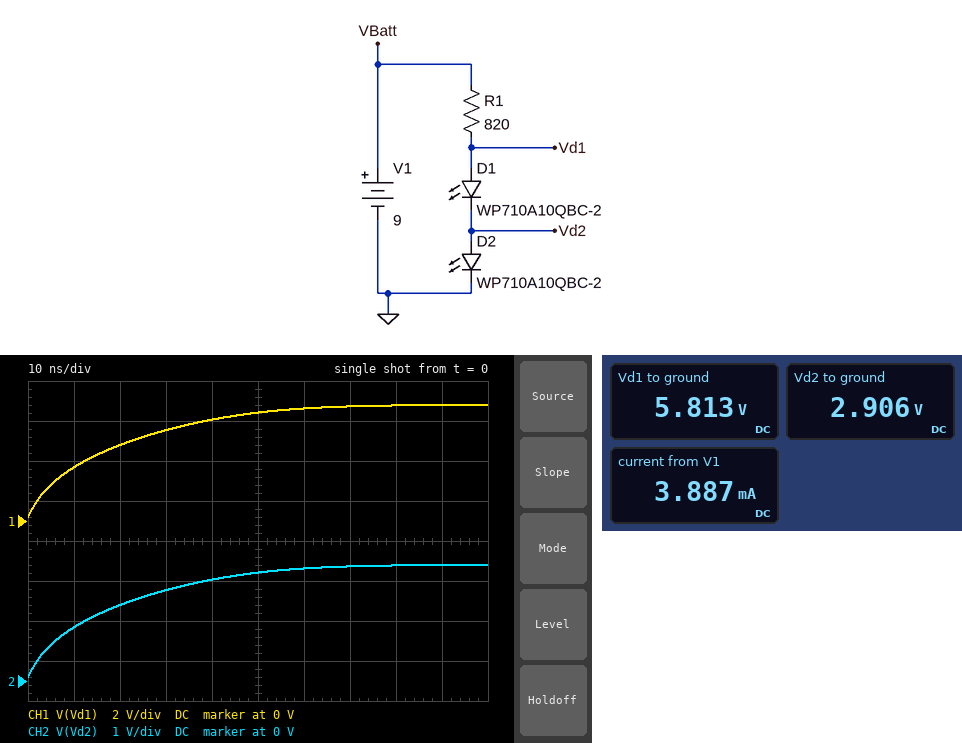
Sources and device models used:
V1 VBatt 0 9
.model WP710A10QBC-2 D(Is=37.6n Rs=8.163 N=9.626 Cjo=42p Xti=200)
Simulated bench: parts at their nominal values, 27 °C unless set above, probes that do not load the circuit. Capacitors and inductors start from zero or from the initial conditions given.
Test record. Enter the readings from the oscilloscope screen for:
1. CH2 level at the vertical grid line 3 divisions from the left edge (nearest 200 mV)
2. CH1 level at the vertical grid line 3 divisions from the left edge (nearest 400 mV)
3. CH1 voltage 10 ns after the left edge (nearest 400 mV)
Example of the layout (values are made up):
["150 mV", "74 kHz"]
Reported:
["2.2 V", "4.4 V", "2.8 V"]
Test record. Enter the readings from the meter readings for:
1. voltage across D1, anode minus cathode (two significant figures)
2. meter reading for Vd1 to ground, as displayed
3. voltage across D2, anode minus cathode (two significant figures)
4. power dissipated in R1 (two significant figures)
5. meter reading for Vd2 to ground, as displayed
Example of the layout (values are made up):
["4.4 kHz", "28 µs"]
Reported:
["2.9 V", "5.813 V", "2.9 V", "12 mW", "2.906 V"]
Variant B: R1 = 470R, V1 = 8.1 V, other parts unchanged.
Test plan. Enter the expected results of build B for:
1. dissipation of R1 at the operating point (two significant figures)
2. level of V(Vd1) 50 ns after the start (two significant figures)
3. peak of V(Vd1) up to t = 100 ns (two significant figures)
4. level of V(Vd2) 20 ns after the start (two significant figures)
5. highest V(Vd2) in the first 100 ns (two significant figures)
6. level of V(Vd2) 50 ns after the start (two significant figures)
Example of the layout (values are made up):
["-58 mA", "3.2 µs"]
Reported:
["10 mW", "5.8 V", "5.9 V", "2.3 V", "3.0 V", "2.9 V"]
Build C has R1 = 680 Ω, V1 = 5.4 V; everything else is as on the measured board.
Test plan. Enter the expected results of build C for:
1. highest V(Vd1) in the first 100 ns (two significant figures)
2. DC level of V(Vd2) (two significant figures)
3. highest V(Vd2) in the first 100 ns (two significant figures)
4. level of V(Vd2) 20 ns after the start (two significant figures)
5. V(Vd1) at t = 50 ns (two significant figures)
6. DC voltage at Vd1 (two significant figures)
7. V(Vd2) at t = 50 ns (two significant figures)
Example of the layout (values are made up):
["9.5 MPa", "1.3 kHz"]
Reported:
["4.7 V", "2.5 V", "2.4 V", "1.4 V", "4.1 V", "4.9 V", "2.0 V"]
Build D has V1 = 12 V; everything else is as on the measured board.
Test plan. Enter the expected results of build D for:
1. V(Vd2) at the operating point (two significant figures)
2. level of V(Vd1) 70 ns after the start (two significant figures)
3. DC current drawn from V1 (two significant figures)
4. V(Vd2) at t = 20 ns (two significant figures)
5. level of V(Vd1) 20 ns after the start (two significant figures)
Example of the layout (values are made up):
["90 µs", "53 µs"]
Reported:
["3.1 V", "6.2 V", "7.1 mA", "2.3 V", "4.6 V"]
